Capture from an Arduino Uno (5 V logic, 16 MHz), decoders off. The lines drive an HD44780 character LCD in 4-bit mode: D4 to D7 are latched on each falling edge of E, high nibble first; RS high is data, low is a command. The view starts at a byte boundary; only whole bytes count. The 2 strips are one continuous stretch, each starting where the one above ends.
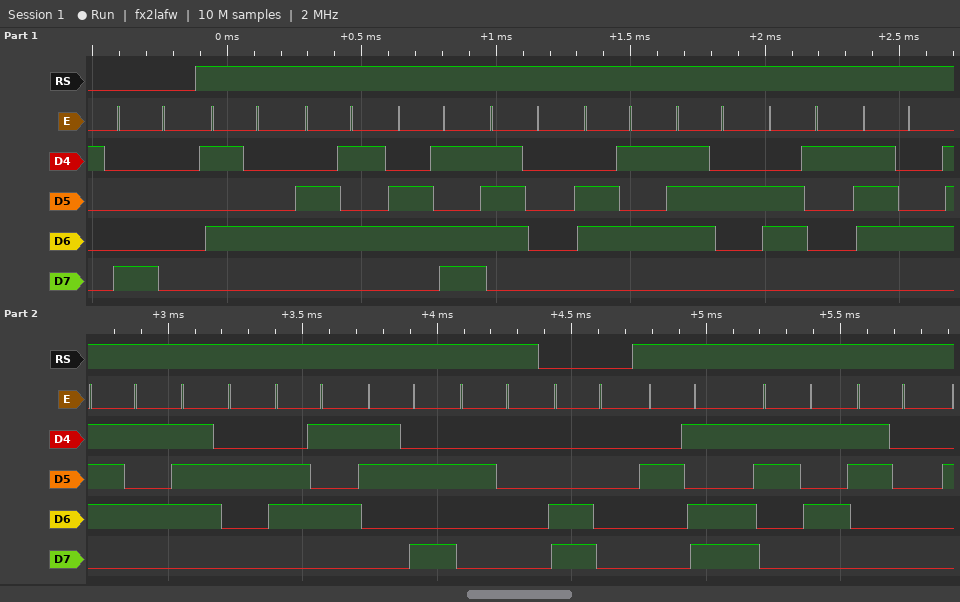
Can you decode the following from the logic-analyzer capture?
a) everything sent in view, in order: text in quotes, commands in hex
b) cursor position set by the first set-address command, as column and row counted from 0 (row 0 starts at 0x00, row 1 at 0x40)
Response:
0x80 "Temperature: " 0xC0 "-50"
column 0, row 0
